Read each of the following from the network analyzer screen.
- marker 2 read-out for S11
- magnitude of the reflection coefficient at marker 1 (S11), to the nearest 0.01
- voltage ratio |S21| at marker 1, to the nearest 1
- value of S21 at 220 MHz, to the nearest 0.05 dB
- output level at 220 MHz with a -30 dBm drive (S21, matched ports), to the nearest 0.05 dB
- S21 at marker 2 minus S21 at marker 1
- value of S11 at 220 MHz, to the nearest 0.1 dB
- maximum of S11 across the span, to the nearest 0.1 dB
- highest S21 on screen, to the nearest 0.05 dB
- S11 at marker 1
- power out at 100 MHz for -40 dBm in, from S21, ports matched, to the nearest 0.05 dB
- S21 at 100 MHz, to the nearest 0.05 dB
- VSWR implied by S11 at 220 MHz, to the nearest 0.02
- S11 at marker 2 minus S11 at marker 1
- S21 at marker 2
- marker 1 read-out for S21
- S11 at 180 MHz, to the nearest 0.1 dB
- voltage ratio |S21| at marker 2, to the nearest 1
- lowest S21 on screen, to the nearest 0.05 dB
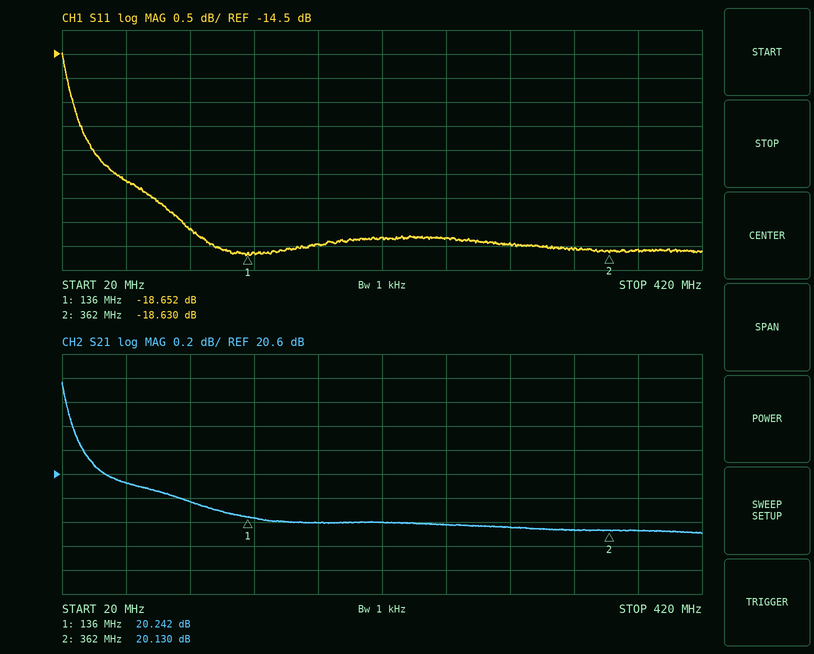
-18.630 dB
0.12
10
20.20 dB
-9.80 dBm
-0.112 dB
-18.3 dB
-14.5 dB
21.35 dB
-18.652 dB
-19.65 dBm
20.35 dB
1.28
0.022 dB
20.130 dB
20.242 dB
-18.5 dB
10
20.10 dB
